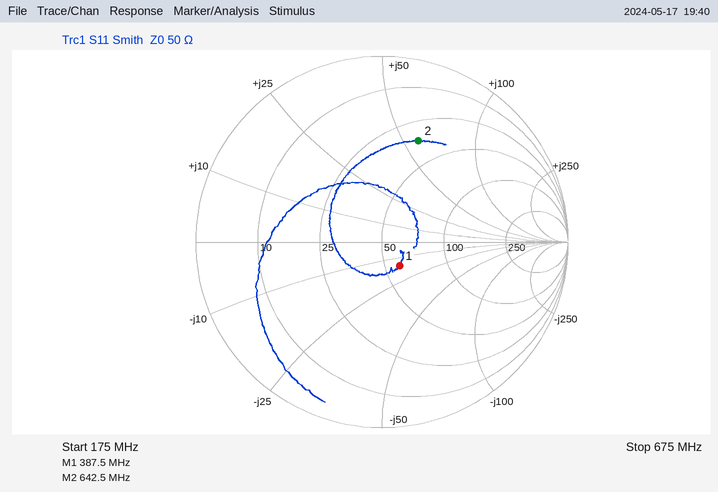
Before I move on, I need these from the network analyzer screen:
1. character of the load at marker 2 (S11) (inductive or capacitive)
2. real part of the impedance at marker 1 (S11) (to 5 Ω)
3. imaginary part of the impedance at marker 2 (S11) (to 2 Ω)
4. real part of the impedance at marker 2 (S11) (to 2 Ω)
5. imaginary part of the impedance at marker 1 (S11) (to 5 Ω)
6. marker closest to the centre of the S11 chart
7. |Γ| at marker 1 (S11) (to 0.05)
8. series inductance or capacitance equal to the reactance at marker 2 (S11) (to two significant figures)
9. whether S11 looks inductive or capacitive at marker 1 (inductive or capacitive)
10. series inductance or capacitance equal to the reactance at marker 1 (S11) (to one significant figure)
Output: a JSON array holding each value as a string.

["inductive", "60 Ω", "+58 Ω", "36 Ω", "-15 Ω", "marker 1", "0.15", "14 nH", "capacitive", "30 pF"]
